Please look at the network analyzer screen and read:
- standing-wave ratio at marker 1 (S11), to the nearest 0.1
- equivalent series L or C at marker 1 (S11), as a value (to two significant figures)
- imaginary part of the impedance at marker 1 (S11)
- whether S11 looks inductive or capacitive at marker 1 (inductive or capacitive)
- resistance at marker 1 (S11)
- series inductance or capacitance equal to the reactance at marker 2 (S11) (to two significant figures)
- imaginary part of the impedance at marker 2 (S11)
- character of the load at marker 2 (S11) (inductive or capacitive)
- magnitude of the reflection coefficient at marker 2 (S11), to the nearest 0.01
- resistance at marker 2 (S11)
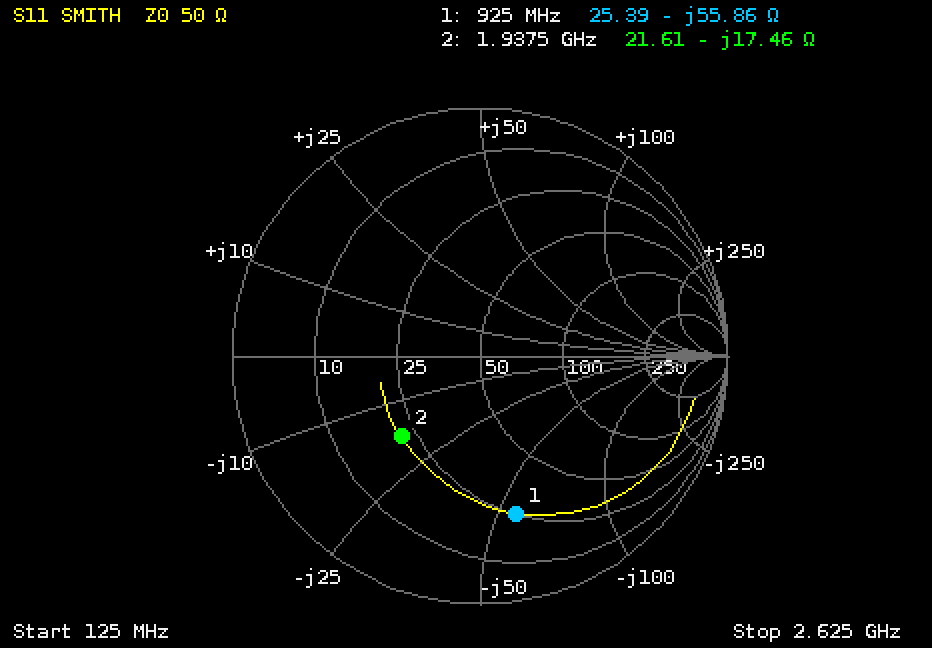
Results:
4.7
3.1 pF
-55.86 Ω
capacitive
25.39 Ω
4.7 pF
-17.46 Ω
capacitive
0.45
21.61 Ω
